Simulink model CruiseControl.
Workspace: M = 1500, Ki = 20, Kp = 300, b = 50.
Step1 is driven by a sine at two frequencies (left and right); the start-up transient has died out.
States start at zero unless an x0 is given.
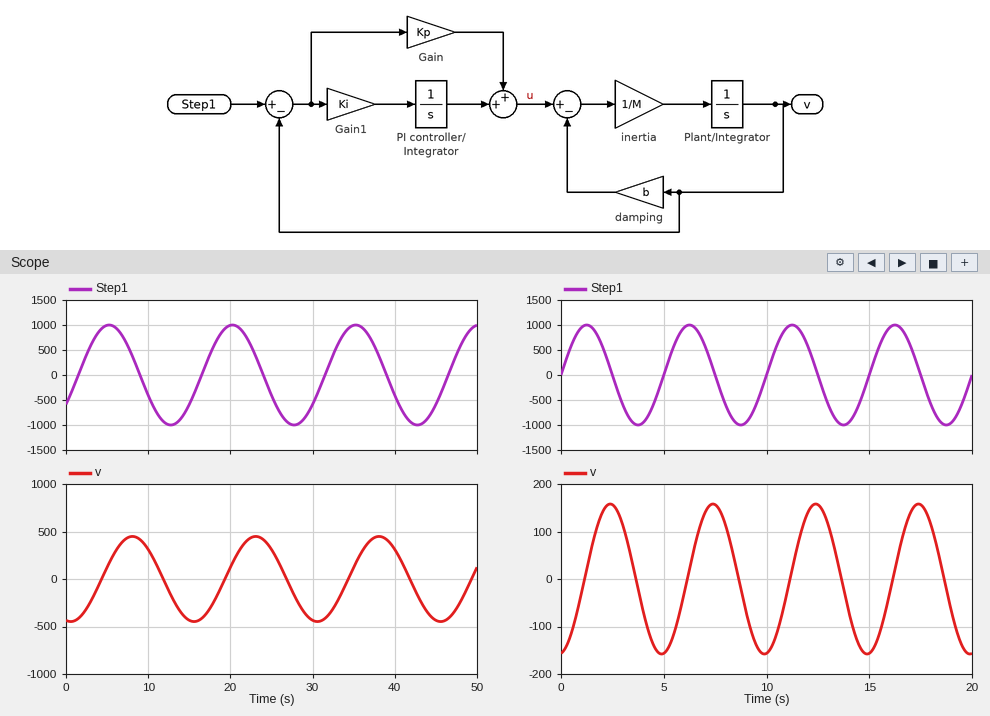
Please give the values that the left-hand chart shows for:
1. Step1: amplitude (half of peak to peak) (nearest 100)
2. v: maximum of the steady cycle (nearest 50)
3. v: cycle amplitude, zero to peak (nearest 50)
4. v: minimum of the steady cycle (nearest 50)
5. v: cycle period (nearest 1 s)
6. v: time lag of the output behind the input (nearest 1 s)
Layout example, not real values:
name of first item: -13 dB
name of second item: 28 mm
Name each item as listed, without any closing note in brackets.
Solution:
Step1: amplitude (half of peak to peak): 1000
v: maximum of the steady cycle: 450
v: cycle amplitude, zero to peak: 450
v: minimum of the steady cycle: -450
v: cycle period: 15 s
v: time lag of the output behind the input: 3 s
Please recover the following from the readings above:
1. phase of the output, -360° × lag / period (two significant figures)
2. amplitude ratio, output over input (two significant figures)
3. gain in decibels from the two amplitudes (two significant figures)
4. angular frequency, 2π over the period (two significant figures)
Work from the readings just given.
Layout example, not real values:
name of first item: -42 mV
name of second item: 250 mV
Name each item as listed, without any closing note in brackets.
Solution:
phase of the output, -360° × lag / period: -72°
amplitude ratio, output over input: 0.45
gain in decibels from the two amplitudes: -6.9 dB
angular frequency, 2π over the period: 0.42 rad/s
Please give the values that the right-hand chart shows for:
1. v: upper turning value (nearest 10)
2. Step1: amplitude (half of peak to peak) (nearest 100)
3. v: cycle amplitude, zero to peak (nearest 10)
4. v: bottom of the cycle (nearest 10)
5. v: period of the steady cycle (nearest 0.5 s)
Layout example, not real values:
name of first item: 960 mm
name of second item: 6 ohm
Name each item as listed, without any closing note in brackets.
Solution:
v: upper turning value: 160
Step1: amplitude (half of peak to peak): 1000
v: cycle amplitude, zero to peak: 160
v: bottom of the cycle: -160
v: period of the steady cycle: 5.0 s
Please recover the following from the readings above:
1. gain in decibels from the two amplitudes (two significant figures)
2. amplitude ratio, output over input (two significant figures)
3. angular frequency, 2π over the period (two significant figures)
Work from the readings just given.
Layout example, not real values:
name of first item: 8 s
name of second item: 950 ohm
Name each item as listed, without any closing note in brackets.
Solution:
gain in decibels from the two amplitudes: -16 dB
amplitude ratio, output over input: 0.16
angular frequency, 2π over the period: 1.3 rad/s
